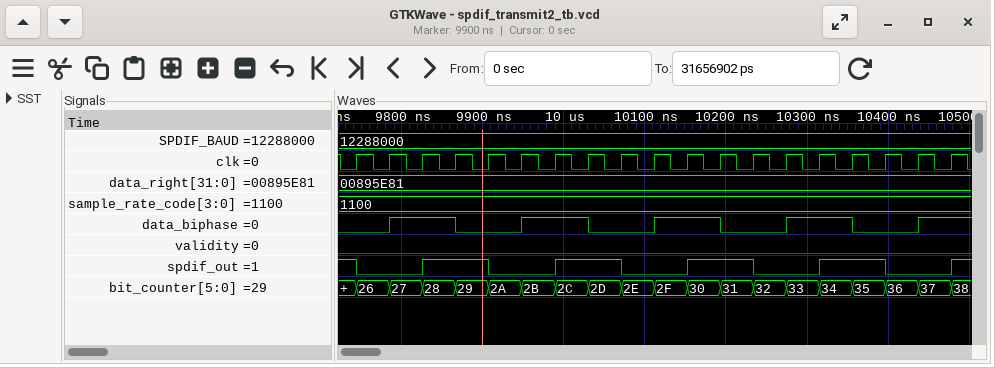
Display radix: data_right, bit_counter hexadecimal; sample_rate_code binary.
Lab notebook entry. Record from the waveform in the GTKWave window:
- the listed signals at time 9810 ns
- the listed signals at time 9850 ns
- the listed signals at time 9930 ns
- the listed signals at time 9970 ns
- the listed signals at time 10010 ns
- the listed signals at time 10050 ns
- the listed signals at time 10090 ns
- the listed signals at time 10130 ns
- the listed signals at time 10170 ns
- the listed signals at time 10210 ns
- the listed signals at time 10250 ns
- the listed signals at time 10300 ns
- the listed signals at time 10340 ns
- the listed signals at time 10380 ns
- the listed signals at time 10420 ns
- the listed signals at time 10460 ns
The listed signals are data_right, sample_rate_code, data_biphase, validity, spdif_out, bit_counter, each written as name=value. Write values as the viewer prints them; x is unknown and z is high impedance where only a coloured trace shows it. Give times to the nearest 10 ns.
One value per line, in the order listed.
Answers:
data_right=00895E81, sample_rate_code=1100, data_biphase=1, validity=0, spdif_out=0, bit_counter=27
data_right=00895E81, sample_rate_code=1100, data_biphase=1, validity=0, spdif_out=1, bit_counter=28
data_right=00895E81, sample_rate_code=1100, data_biphase=0, validity=0, spdif_out=0, bit_counter=2A
data_right=00895E81, sample_rate_code=1100, data_biphase=1, validity=0, spdif_out=0, bit_counter=2B
data_right=00895E81, sample_rate_code=1100, data_biphase=1, validity=0, spdif_out=1, bit_counter=2C
data_right=00895E81, sample_rate_code=1100, data_biphase=0, validity=0, spdif_out=1, bit_counter=2D
data_right=00895E81, sample_rate_code=1100, data_biphase=0, validity=0, spdif_out=0, bit_counter=2E
data_right=00895E81, sample_rate_code=1100, data_biphase=1, validity=0, spdif_out=0, bit_counter=2F
data_right=00895E81, sample_rate_code=1100, data_biphase=1, validity=0, spdif_out=1, bit_counter=30
data_right=00895E81, sample_rate_code=1100, data_biphase=0, validity=0, spdif_out=1, bit_counter=31
data_right=00895E81, sample_rate_code=1100, data_biphase=0, validity=0, spdif_out=0, bit_counter=32
data_right=00895E81, sample_rate_code=1100, data_biphase=1, validity=0, spdif_out=0, bit_counter=33
data_right=00895E81, sample_rate_code=1100, data_biphase=1, validity=0, spdif_out=1, bit_counter=34
data_right=00895E81, sample_rate_code=1100, data_biphase=0, validity=0, spdif_out=1, bit_counter=35
data_right=00895E81, sample_rate_code=1100, data_biphase=0, validity=0, spdif_out=0, bit_counter=36
data_right=00895E81, sample_rate_code=1100, data_biphase=1, validity=0, spdif_out=0, bit_counter=37
